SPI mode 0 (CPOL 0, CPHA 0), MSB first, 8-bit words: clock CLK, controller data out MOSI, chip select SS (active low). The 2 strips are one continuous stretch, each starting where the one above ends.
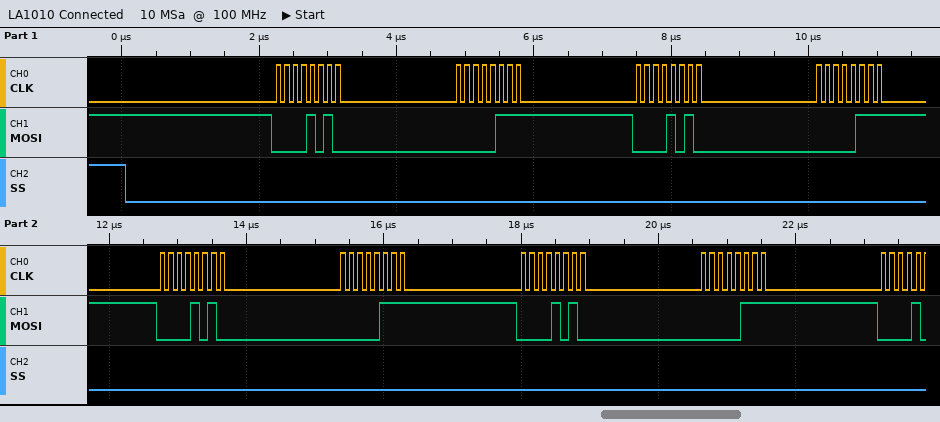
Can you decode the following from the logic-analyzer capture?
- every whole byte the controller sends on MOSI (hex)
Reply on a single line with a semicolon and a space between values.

0A 07 0A 07 0A 07 0A 07
